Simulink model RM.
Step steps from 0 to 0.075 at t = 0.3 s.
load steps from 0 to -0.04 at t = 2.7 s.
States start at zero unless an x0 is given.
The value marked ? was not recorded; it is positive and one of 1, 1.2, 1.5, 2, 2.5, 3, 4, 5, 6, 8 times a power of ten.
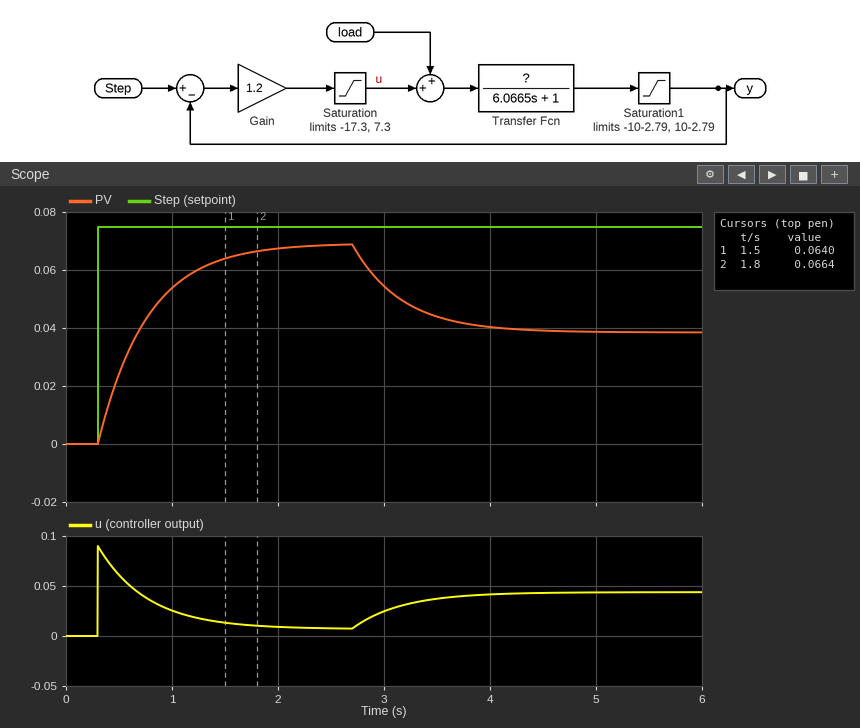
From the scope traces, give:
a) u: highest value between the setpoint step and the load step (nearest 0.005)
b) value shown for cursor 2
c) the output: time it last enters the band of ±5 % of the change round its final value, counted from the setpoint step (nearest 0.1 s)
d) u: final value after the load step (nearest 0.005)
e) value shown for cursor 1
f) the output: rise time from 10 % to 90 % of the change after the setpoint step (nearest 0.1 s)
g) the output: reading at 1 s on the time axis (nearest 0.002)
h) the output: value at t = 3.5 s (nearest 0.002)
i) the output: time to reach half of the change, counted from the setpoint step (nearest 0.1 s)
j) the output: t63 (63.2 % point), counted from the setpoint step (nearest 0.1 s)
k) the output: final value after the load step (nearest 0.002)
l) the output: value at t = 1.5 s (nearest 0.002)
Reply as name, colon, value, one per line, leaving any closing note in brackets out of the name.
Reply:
u: highest value between the setpoint step and the load step: 0.090
value shown for cursor 2: 0.0664
the output: time it last enters the band of ±5 % of the change round its final value, counted from the setpoint step: 1.4 s
u: final value after the load step: 0.045
value shown for cursor 1: 0.0640
the output: rise time from 10 % to 90 % of the change after the setpoint step: 1.0 s
the output: reading at 1 s on the time axis: 0.054
the output: value at t = 3.5 s: 0.044
the output: time to reach half of the change, counted from the setpoint step: 0.3 s
the output: t63 (63.2 % point), counted from the setpoint step: 0.5 s
the output: final value after the load step: 0.038
the output: value at t = 1.5 s: 0.064
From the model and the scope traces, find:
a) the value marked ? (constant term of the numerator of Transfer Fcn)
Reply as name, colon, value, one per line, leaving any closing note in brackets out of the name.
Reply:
the value marked ?: 10
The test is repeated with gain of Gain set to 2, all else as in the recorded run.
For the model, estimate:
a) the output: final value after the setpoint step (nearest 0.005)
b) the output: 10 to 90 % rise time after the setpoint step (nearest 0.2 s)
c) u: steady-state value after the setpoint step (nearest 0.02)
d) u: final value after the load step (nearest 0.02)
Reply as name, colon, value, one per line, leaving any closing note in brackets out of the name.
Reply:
the output: final value after the setpoint step: 0.070
the output: 10 to 90 % rise time after the setpoint step: 0.6 s
u: steady-state value after the setpoint step: 0.00
u: final value after the load step: 0.04
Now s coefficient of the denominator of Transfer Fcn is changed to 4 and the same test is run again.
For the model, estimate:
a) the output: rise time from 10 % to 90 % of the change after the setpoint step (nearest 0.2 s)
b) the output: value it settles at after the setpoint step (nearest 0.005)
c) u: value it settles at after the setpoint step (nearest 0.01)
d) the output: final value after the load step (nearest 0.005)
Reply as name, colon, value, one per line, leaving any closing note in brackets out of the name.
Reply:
the output: rise time from 10 % to 90 % of the change after the setpoint step: 0.6 s
the output: value it settles at after the setpoint step: 0.070
u: value it settles at after the setpoint step: 0.01
the output: final value after the load step: 0.040
